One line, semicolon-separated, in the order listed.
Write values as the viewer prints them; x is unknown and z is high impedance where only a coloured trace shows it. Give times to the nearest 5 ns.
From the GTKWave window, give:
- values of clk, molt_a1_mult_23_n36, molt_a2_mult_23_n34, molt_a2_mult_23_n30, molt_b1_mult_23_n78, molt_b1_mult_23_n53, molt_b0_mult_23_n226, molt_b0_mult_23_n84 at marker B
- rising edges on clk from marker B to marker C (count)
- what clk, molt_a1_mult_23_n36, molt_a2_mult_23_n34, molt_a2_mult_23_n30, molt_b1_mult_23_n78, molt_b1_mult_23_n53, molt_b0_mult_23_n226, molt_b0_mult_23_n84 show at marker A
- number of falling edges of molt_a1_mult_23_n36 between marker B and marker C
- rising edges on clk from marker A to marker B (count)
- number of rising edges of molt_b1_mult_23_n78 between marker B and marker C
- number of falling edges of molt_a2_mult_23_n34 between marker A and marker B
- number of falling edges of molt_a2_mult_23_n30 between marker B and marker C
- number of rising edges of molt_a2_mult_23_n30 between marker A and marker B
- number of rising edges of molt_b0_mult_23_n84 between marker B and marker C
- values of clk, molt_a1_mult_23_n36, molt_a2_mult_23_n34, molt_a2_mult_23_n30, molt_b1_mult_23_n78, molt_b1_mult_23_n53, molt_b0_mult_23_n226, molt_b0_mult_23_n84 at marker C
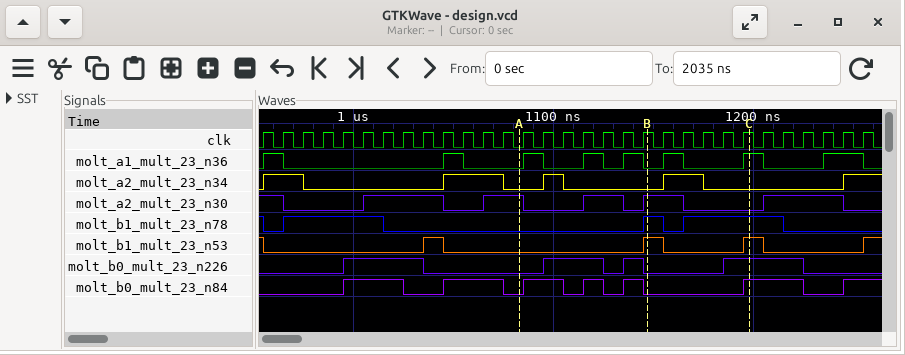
clk=1, molt_a1_mult_23_n36=0, molt_a2_mult_23_n34=0, molt_a2_mult_23_n30=1, molt_b1_mult_23_n78=1, molt_b1_mult_23_n53=1, molt_b0_mult_23_n226=0, molt_b0_mult_23_n84=0; 5; clk=0, molt_a1_mult_23_n36=0, molt_a2_mult_23_n34=0, molt_a2_mult_23_n30=1, molt_b1_mult_23_n78=0, molt_b1_mult_23_n53=0, molt_b0_mult_23_n226=0, molt_b0_mult_23_n84=0; 1; 7; 1; 1; 1; 2; 1; clk=1, molt_a1_mult_23_n36=1, molt_a2_mult_23_n34=0, molt_a2_mult_23_n30=0, molt_b1_mult_23_n78=1, molt_b1_mult_23_n53=1, molt_b0_mult_23_n226=1, molt_b0_mult_23_n84=1
